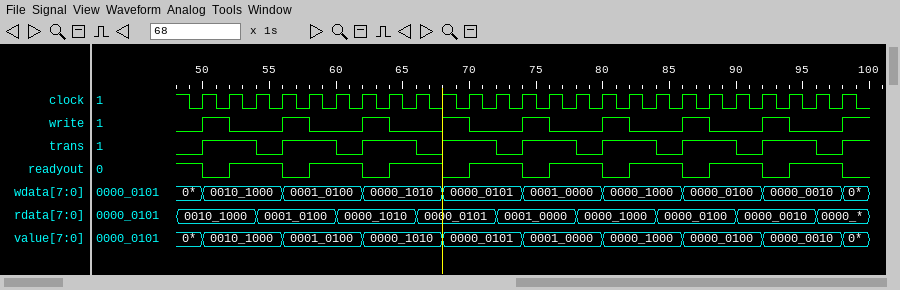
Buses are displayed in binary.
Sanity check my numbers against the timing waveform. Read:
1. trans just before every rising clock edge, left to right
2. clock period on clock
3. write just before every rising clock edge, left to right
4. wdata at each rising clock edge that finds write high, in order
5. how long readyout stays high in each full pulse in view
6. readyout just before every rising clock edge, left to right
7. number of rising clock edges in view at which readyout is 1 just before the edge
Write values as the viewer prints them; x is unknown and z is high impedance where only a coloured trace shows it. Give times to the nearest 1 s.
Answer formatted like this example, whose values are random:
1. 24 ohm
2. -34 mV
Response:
1. 0 1 1 0 1 1 0 1 1 0 1 1 0 1 1 0 1 1 0 1 1 0 1 1 0
2. 2 s
3. 0 1 0 0 1 0 0 1 0 0 1 0 0 1 0 0 1 0 0 1 0 0 1 0 0
4. 0010_1000, 0001_0100, 0000_1010, 0000_0101, 0001_0000, 0000_1000, 0000_0100, 0000_0010
5. 4 s, 4 s, 4 s, 4 s, 4 s, 4 s, 4 s, 4 s
6. 1 0 1 1 0 1 1 0 1 1 0 1 1 0 1 1 0 1 1 0 1 1 0 1 1
7. 17
